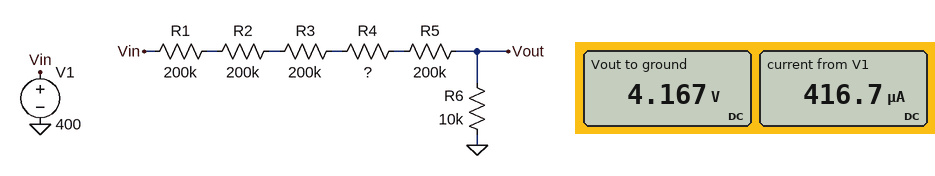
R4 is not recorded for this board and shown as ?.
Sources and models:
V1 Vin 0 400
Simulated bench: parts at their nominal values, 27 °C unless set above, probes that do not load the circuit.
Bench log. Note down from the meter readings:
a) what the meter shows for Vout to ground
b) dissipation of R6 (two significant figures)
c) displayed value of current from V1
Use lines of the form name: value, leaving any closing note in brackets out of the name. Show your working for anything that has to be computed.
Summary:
what the meter shows for Vout to ground: 4.167 V
dissipation of R6: (4.167 V)^2 / 10 kΩ = 1.7 mW
displayed value of current from V1: 416.7 µA
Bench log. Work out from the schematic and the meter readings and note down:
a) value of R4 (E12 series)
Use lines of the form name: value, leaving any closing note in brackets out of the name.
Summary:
value of R4: 150 kΩ
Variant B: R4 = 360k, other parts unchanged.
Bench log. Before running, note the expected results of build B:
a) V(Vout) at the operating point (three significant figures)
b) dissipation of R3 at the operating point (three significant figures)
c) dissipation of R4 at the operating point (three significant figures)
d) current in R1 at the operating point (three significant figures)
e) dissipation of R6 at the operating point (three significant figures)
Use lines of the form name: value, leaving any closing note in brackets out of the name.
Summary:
V(Vout) at the operating point: 3.42 V
dissipation of R3 at the operating point: 23.4 mW
dissipation of R4 at the operating point: 42.1 mW
current in R1 at the operating point: 342 µA
dissipation of R6 at the operating point: 1.17 mW
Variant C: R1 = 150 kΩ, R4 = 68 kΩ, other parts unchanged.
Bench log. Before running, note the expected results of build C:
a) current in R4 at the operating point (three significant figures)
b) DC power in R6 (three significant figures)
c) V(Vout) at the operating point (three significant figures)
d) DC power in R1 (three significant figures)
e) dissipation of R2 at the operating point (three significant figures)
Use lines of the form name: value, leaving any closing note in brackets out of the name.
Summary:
current in R4 at the operating point: 483 µA
DC power in R6: 2.33 mW
V(Vout) at the operating point: 4.83 V
DC power in R1: 35.0 mW
dissipation of R2 at the operating point: 46.7 mW
